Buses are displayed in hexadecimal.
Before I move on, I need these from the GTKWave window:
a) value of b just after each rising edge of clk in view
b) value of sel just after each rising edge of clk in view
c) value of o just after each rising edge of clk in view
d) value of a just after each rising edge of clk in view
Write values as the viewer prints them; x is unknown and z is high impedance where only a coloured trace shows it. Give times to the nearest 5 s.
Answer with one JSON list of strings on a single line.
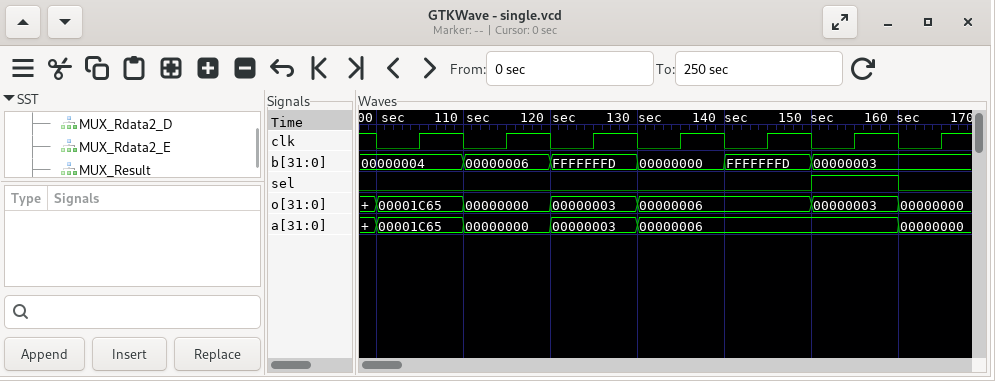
["00000004, 00000006, FFFFFFFD, 00000000, FFFFFFFD, 00000003, 00000003", "0 0 0 0 0 1 0", "00001C65, 00000000, 00000003, 00000006, 00000006, 00000003, 00000000", "00001C65, 00000000, 00000003, 00000006, 00000006, 00000006, 00000000"]
